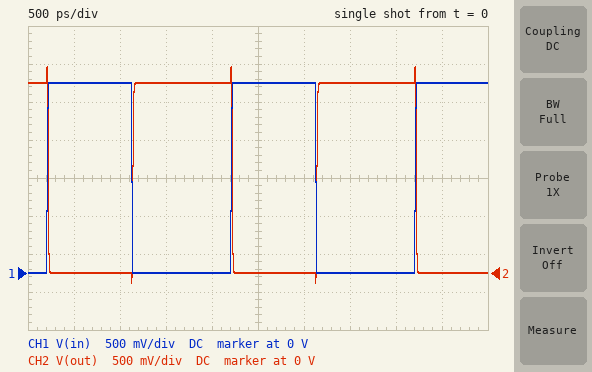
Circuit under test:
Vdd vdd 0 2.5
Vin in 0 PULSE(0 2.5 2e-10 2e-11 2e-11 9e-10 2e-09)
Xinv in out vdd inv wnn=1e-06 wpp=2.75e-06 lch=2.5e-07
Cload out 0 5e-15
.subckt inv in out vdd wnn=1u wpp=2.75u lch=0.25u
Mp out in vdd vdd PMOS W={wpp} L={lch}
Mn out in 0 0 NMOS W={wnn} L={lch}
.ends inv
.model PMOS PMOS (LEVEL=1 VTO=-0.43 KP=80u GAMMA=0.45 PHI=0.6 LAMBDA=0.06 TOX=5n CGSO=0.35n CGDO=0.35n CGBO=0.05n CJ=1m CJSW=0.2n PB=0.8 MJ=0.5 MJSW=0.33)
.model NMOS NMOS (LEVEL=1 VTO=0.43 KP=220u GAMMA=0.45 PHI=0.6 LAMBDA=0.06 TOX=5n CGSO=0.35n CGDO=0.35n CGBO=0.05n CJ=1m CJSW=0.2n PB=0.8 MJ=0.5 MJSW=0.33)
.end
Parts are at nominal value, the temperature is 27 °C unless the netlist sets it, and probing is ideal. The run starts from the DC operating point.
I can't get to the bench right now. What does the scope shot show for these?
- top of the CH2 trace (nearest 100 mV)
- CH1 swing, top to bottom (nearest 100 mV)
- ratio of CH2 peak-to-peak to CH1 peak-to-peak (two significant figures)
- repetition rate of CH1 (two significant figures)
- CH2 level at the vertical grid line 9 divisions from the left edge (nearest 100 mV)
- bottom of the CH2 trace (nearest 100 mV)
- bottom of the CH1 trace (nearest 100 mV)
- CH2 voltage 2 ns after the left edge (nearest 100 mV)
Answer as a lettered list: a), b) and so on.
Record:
a) 2.7 V
b) 2.5 V
c) 1.1
d) 500 MHz
e) 0 V
f) -100 mV
g) 0 V
h) 2.5 V
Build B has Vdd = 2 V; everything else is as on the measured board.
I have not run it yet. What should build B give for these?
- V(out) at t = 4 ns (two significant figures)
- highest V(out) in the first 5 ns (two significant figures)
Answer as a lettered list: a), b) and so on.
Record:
a) 2.0 V
b) 2.3 V
